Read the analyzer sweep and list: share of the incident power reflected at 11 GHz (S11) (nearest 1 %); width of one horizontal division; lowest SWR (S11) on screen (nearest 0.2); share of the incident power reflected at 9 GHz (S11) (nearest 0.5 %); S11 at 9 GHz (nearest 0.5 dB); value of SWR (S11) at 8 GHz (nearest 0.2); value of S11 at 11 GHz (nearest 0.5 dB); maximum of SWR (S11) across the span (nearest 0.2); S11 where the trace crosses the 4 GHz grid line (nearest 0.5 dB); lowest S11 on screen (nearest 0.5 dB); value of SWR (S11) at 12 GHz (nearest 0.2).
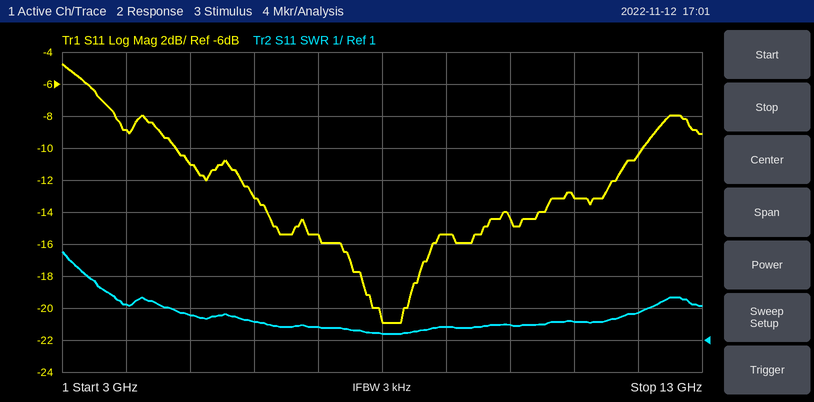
5 %
1 GHz
1.2
3.0 %
-15.5 dB
1.2
-13.0 dB
3.8
-9.0 dB
-21.0 dB
1.8
